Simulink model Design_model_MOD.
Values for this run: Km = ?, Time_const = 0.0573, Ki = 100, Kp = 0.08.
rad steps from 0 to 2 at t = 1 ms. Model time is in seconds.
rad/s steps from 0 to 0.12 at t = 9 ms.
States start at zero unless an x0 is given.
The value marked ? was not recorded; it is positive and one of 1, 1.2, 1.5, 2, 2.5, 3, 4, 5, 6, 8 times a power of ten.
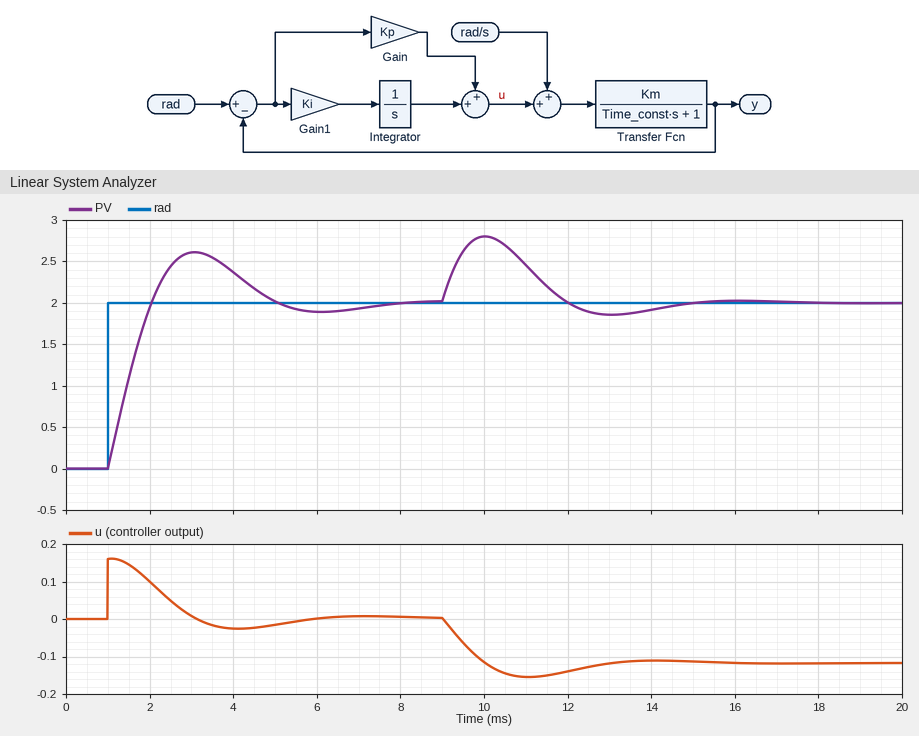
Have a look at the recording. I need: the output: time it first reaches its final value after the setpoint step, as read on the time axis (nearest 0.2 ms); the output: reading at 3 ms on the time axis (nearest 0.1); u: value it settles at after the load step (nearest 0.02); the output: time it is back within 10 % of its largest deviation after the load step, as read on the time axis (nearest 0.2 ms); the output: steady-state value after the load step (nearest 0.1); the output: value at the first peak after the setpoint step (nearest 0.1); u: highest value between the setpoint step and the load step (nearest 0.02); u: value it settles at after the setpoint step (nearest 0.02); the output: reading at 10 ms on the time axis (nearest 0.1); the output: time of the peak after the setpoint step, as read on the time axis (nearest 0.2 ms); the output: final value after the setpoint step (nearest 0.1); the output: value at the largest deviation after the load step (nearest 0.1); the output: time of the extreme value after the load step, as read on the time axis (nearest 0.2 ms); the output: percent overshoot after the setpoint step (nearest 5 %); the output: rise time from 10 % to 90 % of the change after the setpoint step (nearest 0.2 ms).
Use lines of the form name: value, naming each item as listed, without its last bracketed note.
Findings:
the output: time it first reaches its final value after the setpoint step, as read on the time axis: 2.0 ms
the output: reading at 3 ms on the time axis: 2.6
u: value it settles at after the load step: -0.12
the output: time it is back within 10 % of its largest deviation after the load step, as read on the time axis: 14.0 ms
the output: steady-state value after the load step: 2.0
the output: value at the first peak after the setpoint step: 2.6
u: highest value between the setpoint step and the load step: 0.16
u: value it settles at after the setpoint step: 0.00
the output: reading at 10 ms on the time axis: 2.8
the output: time of the peak after the setpoint step, as read on the time axis: 3.0 ms
the output: final value after the setpoint step: 2.0
the output: value at the largest deviation after the load step: 2.8
the output: time of the extreme value after the load step, as read on the time axis: 10.0 ms
the output: percent overshoot after the setpoint step: 30 %
the output: rise time from 10 % to 90 % of the change after the setpoint step: 0.8 ms
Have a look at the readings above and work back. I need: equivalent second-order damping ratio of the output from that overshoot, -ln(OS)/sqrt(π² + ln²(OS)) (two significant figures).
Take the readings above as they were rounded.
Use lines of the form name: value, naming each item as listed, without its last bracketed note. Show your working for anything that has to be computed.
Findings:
equivalent second-order damping ratio of the output from that overshoot, -ln(OS)/sqrt(π² + ln²(OS)): ln(0.3) = -1.204; 1.204 / sqrt(9.870 + 1.450) = 0.36
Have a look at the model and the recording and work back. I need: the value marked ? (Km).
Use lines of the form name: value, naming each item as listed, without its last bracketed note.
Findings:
the value marked ?: 800
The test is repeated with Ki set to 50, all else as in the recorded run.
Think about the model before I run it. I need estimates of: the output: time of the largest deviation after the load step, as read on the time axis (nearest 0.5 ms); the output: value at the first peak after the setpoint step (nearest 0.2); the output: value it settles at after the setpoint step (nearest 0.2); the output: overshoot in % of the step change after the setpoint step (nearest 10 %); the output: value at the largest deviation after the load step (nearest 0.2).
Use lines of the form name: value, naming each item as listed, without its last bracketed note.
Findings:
the output: time of the largest deviation after the load step, as read on the time axis: 10.5 ms
the output: value at the first peak after the setpoint step: 2.4
the output: value it settles at after the setpoint step: 2.0
the output: overshoot in % of the step change after the setpoint step: 20 %
the output: value at the largest deviation after the load step: 3.0
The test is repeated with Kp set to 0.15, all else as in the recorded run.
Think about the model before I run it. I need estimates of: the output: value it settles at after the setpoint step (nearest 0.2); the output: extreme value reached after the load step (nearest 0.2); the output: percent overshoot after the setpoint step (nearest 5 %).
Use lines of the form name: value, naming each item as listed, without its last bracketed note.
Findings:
the output: value it settles at after the setpoint step: 2.0
the output: extreme value reached after the load step: 2.6
the output: percent overshoot after the setpoint step: 15 %
